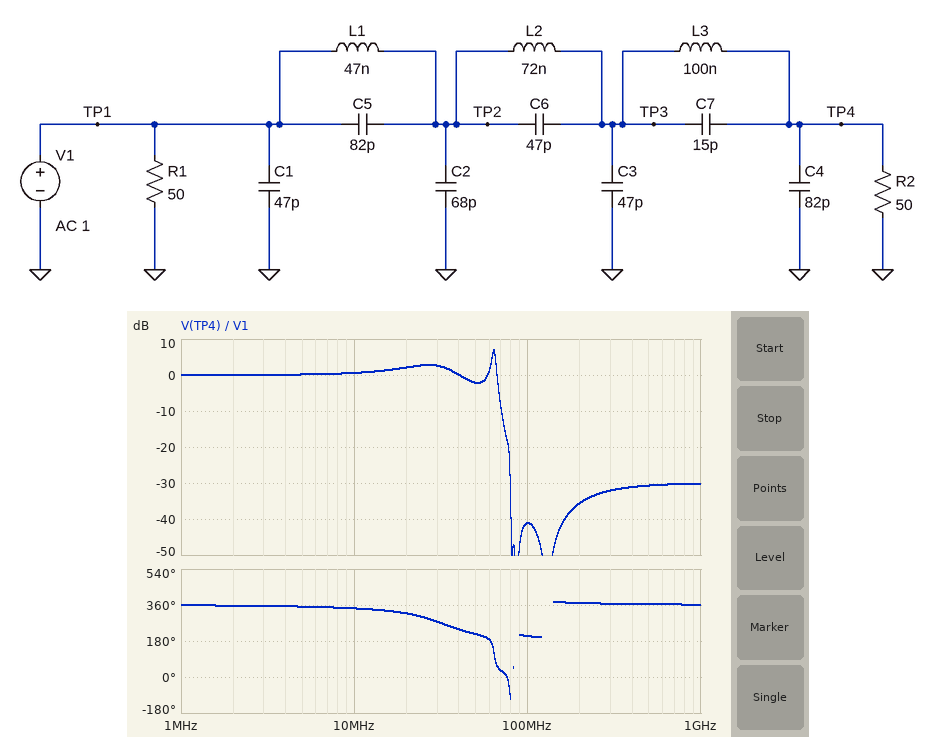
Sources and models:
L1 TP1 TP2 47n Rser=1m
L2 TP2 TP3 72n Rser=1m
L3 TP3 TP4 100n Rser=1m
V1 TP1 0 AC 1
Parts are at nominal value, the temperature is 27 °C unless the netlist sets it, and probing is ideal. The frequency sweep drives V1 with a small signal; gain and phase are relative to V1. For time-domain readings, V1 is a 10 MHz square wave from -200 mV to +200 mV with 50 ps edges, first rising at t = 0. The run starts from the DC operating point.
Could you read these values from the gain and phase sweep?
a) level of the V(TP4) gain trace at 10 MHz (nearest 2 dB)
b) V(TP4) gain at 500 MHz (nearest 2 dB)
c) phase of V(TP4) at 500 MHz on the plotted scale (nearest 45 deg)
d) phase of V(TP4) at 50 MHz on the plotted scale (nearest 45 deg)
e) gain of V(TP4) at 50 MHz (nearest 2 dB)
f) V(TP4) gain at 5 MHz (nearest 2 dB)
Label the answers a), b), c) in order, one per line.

a) 0 dB
b) -30 dB
c) 360 deg
d) 225 deg
e) -2 dB
f) 0 dB
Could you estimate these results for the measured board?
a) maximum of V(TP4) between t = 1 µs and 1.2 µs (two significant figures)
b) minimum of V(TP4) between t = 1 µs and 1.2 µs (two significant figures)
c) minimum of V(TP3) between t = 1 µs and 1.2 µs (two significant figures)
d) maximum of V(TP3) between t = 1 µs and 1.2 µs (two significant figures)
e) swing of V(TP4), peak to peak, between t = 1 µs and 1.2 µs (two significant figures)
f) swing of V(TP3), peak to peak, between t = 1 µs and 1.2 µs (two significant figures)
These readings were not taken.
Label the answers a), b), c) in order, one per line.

a) 330 mV
b) -330 mV
c) -270 mV
d) 270 mV
e) 660 mV
f) 540 mV
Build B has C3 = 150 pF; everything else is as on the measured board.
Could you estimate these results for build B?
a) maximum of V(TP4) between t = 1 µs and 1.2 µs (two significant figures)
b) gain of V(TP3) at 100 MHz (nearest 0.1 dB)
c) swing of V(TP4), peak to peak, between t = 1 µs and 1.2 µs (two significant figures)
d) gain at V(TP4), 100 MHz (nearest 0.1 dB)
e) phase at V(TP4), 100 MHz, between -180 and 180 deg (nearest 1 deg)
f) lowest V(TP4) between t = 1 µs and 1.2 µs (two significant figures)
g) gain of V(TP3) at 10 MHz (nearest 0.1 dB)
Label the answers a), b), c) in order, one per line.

a) 400 mV
b) -33.7 dB
c) 790 mV
d) -51.3 dB
e) -156 deg
f) -400 mV
g) 0.8 dB
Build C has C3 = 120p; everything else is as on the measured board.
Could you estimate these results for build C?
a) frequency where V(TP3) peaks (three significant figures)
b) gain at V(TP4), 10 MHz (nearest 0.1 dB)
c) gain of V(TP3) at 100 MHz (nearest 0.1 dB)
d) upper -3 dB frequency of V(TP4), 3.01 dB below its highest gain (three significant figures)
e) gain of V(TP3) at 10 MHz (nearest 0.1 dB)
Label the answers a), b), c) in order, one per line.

a) 69.7 MHz
b) 0.9 dB
c) -31.7 dB
d) 70.2 MHz
e) 0.7 dB
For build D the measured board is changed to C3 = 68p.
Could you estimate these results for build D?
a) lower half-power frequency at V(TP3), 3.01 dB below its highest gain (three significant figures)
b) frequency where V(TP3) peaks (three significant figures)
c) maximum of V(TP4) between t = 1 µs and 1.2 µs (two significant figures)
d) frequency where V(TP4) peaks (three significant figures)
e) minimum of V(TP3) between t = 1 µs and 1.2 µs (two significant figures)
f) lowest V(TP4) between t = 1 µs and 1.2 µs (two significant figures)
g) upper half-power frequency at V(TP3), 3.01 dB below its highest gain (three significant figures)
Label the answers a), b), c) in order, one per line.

a) 60.3 MHz
b) 63.1 MHz
c) 350 mV
d) 62.8 MHz
e) -290 mV
f) -350 mV
g) 65.9 MHz
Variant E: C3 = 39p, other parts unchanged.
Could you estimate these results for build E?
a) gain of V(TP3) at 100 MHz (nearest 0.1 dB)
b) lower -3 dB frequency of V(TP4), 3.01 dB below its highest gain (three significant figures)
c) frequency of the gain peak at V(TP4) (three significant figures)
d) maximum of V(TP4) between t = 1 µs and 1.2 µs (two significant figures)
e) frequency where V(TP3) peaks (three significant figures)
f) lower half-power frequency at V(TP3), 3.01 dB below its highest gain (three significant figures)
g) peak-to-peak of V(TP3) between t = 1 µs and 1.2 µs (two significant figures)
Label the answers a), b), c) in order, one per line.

a) -21.8 dB
b) 62.6 MHz
c) 64.2 MHz
d) 320 mV
e) 64.3 MHz
f) 62.9 MHz
g) 530 mV
